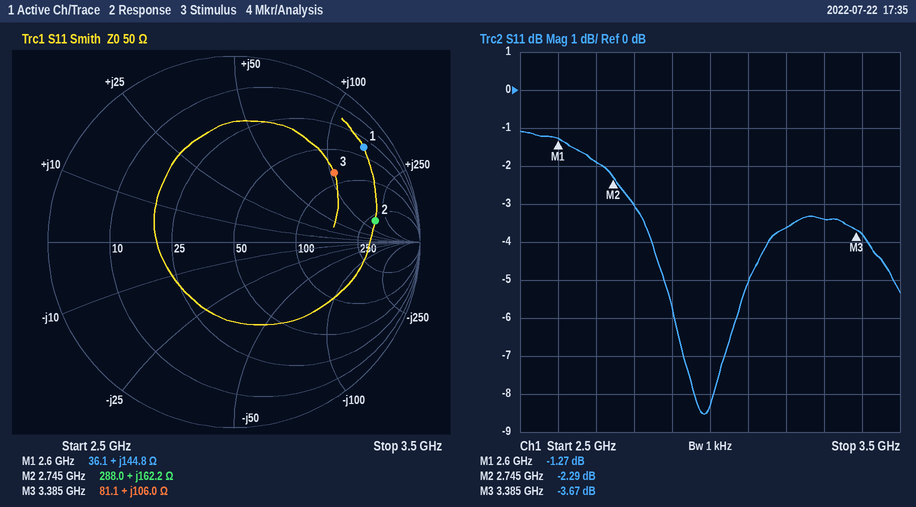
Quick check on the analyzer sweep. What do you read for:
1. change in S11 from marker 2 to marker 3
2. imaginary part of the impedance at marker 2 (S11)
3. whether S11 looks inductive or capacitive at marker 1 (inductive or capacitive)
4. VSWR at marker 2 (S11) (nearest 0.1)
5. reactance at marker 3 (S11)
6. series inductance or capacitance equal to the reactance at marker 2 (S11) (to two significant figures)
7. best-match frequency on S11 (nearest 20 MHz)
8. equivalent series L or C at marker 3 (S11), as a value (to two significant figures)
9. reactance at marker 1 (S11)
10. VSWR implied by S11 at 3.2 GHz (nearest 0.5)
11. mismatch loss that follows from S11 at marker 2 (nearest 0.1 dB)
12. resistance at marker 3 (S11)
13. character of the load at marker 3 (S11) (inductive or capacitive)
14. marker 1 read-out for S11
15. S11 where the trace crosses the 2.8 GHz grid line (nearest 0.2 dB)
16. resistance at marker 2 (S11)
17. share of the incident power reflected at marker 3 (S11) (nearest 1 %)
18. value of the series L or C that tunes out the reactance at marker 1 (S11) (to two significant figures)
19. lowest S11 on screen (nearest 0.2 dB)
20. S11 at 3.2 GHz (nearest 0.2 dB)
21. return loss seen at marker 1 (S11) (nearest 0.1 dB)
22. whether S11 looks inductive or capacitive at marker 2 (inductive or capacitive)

-1.38 dB
+162.2 Ω
inductive
7.6
+106.0 Ω
9.4 nH
2.98 GHz
5.0 nH
+144.8 Ω
5.0
3.9 dB
81.1 Ω
inductive
-1.27 dB
-3.0 dB
288.0 Ω
43 %
420 fF
-8.6 dB
-3.6 dB
1.3 dB
inductive
